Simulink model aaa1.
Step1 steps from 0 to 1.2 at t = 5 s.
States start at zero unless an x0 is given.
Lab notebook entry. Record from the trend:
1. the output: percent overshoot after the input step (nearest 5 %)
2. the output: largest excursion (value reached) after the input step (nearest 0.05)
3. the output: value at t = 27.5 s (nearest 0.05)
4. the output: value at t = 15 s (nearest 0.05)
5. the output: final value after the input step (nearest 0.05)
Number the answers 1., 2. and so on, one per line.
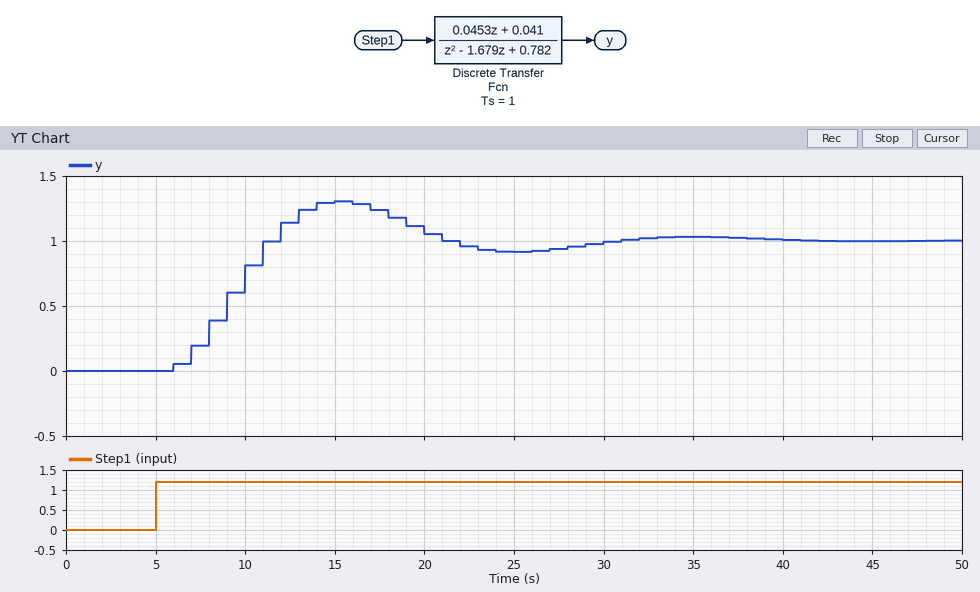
1. 30 %
2. 1.30
3. 0.95
4. 1.30
5. 1.00
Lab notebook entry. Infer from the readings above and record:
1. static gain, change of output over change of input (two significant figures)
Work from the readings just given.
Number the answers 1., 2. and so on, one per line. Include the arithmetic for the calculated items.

1. (1 - 0) / (1.2 - 0) = 0.83
